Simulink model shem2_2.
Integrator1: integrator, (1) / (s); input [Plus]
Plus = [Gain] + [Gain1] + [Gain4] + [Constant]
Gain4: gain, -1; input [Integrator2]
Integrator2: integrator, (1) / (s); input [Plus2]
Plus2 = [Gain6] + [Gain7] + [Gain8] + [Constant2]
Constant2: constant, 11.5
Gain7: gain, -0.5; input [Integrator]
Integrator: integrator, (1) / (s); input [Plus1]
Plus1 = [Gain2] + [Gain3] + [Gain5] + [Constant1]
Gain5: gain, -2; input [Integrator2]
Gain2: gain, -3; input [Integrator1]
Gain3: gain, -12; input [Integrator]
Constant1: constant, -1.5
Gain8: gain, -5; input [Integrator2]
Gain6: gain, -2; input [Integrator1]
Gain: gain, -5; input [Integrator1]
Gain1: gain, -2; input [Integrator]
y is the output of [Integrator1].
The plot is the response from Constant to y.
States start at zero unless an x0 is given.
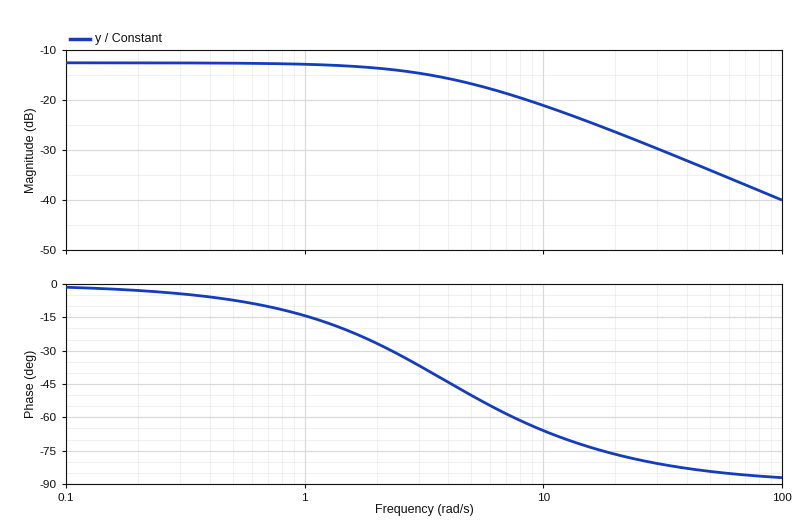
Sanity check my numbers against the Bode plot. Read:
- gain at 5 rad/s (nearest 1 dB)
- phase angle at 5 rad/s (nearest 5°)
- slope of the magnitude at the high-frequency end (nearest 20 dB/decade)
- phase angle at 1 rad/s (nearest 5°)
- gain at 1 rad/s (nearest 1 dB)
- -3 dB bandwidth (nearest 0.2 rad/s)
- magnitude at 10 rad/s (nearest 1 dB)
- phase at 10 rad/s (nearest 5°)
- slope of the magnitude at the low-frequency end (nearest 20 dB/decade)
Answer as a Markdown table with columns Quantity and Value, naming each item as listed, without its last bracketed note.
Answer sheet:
| Quantity | Value |
|---|---|
| gain at 5 rad/s | -17 dB |
| phase angle at 5 rad/s | -50° |
| slope of the magnitude at the high-frequency end | -20 dB/decade |
| phase angle at 1 rad/s | -15° |
| gain at 1 rad/s | -13 dB |
| -3 dB bandwidth | 3.8 rad/s |
| magnitude at 10 rad/s | -21 dB |
| phase at 10 rad/s | -65° |
| slope of the magnitude at the low-frequency end | 0 dB/decade |
